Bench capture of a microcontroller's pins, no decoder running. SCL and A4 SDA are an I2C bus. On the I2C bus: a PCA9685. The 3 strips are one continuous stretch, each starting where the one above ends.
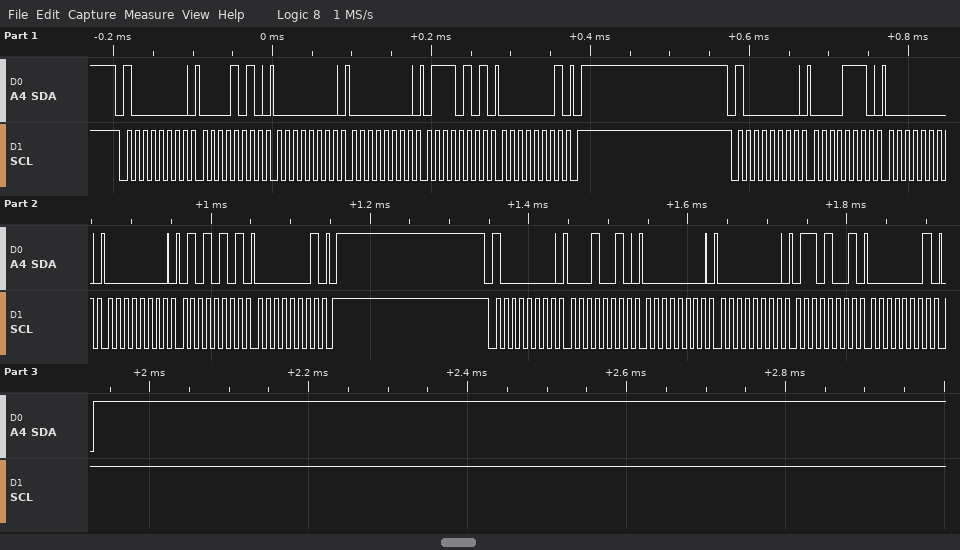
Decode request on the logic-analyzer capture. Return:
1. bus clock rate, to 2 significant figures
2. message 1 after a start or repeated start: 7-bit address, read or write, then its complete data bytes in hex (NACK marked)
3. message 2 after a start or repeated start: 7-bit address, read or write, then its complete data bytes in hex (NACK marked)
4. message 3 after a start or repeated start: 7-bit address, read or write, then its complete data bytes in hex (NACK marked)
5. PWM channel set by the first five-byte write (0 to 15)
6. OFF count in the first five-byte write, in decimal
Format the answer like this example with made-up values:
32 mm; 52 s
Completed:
100 kHz; 0x40 write: 0A 00 00 75 01; 0x40 write: 0E 00 00 55 01; 0x40 write: 12 00 00 69 01; 1; 373
